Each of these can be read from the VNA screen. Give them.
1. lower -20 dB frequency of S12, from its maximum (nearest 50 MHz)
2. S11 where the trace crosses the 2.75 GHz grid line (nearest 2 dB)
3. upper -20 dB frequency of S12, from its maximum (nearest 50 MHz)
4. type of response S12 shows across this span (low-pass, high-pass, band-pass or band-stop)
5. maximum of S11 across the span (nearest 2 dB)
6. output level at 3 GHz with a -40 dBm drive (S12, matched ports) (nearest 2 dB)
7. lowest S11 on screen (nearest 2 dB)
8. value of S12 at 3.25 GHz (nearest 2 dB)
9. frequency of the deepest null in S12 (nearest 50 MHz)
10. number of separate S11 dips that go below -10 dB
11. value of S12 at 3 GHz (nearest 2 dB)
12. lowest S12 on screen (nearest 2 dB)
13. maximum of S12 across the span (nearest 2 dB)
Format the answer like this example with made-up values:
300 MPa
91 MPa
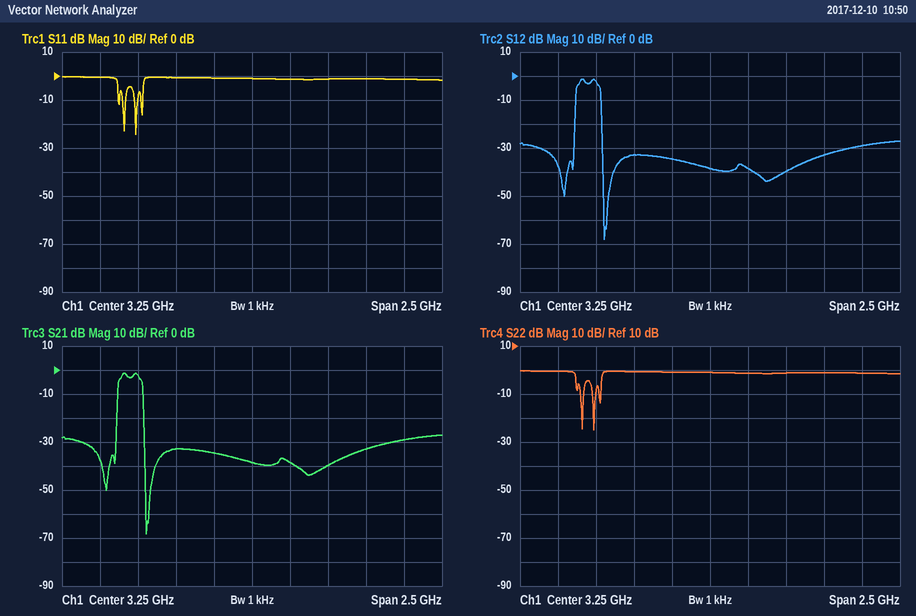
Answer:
2.35 GHz
0 dB
2.55 GHz
band-pass
0 dB
-74 dBm
-24 dB
-38 dB
2.55 GHz
4
-34 dB
-68 dB
-2 dB
